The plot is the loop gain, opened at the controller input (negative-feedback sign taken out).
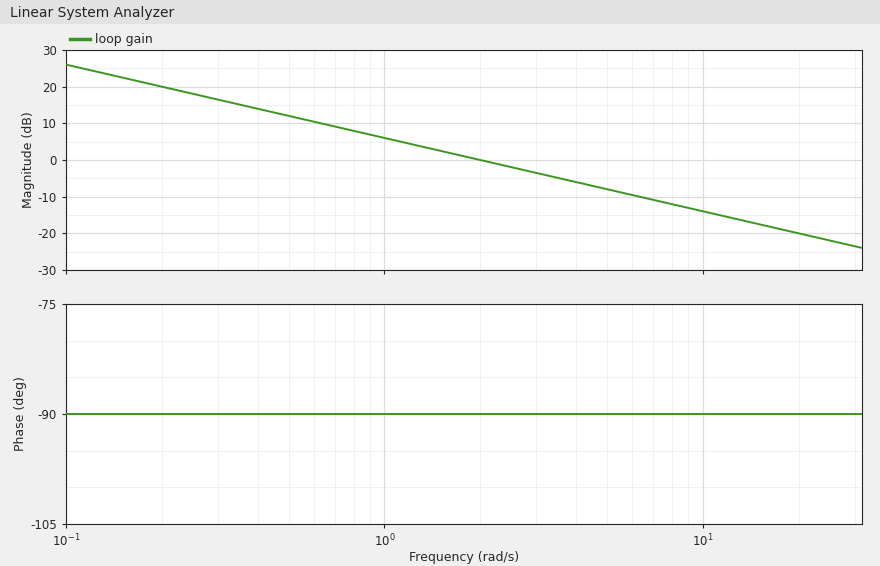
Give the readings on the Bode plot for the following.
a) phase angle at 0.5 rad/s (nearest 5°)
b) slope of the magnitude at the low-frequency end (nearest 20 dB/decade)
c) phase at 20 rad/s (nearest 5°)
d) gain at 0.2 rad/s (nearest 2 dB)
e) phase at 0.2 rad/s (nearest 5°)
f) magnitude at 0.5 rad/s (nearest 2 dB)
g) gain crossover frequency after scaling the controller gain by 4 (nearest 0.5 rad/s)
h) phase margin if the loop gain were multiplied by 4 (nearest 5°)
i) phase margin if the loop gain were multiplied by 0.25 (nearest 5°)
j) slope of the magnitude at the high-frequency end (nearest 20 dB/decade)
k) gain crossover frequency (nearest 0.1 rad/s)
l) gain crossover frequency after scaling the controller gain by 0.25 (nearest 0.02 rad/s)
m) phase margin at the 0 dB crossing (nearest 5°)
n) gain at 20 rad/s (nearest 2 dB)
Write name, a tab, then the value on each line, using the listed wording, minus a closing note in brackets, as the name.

phase angle at 0.5 rad/s	-90°
slope of the magnitude at the low-frequency end	-20 dB/decade
phase at 20 rad/s	-90°
gain at 0.2 rad/s	20 dB
phase at 0.2 rad/s	-90°
magnitude at 0.5 rad/s	12 dB
gain crossover frequency after scaling the controller gain by 4	8.0 rad/s
phase margin if the loop gain were multiplied by 4	90°
phase margin if the loop gain were multiplied by 0.25	90°
slope of the magnitude at the high-frequency end	-20 dB/decade
gain crossover frequency	2.0 rad/s
gain crossover frequency after scaling the controller gain by 0.25	0.50 rad/s
phase margin at the 0 dB crossing	90°
gain at 20 rad/s	-20 dB
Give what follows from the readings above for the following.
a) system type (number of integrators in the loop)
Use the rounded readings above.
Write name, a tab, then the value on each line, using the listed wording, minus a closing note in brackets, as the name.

system type	1
